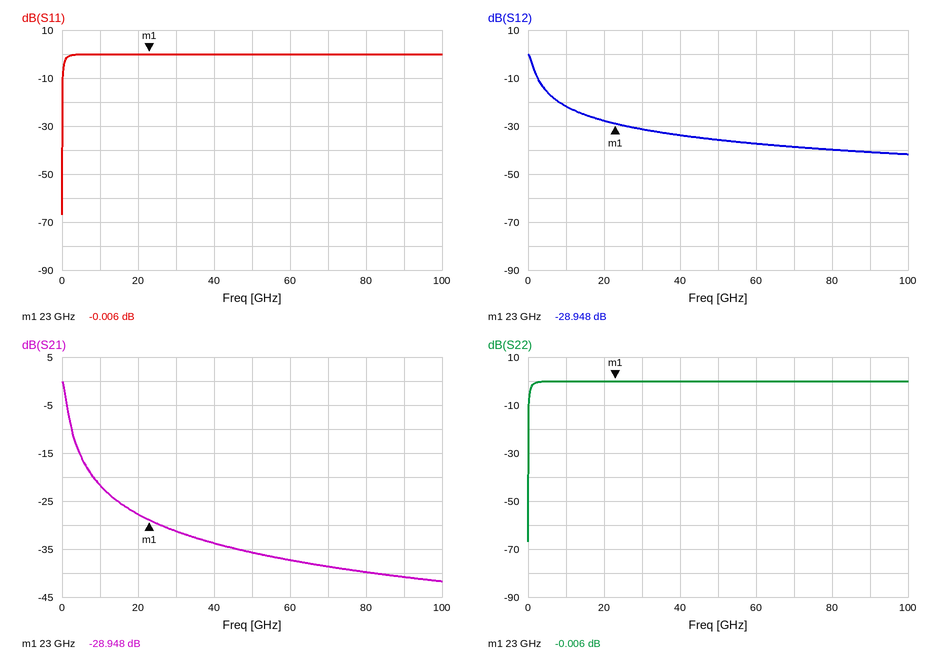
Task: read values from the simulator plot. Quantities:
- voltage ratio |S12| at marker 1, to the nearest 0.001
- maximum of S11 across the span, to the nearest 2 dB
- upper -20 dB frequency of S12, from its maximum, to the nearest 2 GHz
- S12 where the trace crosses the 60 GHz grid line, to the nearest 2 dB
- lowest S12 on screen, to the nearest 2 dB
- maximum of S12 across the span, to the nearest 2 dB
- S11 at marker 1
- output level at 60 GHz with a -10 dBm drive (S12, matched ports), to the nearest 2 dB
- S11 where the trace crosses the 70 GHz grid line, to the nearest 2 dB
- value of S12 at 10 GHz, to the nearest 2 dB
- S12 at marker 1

0.036
0 dB
8 GHz
-38 dB
-42 dB
0 dB
-0.006 dB
-48 dBm
0 dB
-22 dB
-28.948 dB
